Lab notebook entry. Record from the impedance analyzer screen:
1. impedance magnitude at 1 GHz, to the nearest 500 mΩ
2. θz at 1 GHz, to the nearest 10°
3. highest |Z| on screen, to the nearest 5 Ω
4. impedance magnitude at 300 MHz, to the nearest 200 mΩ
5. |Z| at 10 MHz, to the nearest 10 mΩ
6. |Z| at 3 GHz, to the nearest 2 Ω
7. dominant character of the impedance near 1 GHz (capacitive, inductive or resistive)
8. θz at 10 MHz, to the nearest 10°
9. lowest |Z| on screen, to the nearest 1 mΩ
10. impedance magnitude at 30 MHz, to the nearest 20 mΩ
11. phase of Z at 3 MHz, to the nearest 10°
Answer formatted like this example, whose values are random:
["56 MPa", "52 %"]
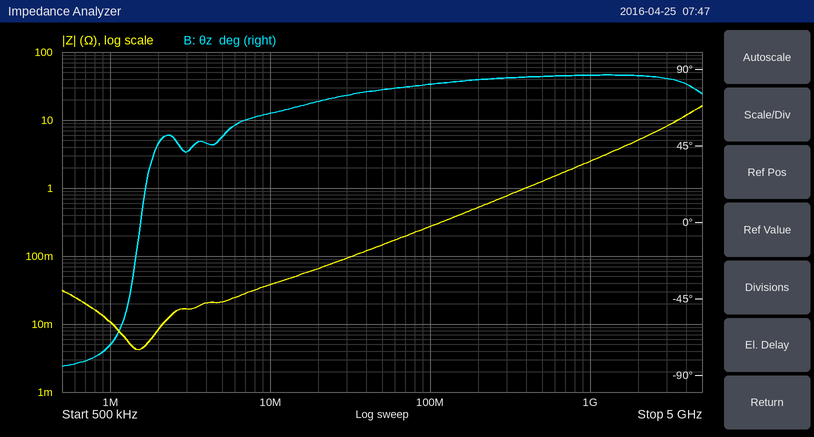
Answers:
["2.5 Ω", "90°", "15 Ω", "800 mΩ", "40 mΩ", "8 Ω", "inductive", "60°", "4 mΩ", "100 mΩ", "40°"]
